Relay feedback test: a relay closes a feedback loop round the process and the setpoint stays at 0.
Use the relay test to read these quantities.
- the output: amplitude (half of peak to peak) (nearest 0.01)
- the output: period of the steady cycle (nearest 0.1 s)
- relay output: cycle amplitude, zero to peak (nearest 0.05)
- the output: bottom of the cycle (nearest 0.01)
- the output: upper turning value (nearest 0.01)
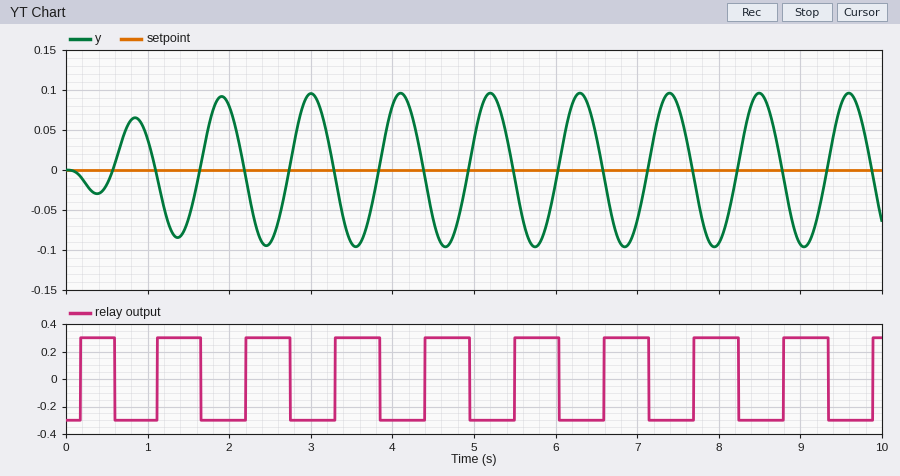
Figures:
0.10
1.1 s
0.30
-0.10
0.10
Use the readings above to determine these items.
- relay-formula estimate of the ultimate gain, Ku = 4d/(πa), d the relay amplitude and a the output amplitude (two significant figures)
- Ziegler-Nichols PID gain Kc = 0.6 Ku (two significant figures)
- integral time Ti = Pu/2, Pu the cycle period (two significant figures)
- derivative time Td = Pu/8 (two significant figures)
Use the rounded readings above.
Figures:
3.8
2.3
0.55 s
0.14 s
